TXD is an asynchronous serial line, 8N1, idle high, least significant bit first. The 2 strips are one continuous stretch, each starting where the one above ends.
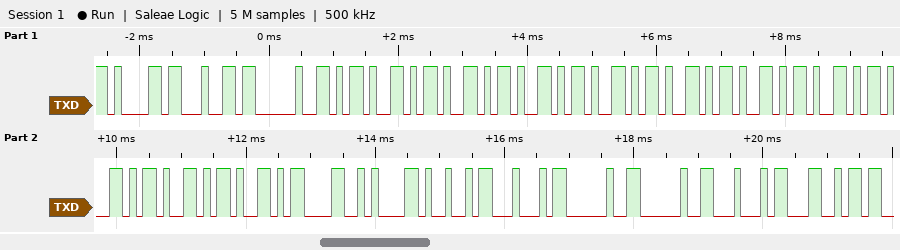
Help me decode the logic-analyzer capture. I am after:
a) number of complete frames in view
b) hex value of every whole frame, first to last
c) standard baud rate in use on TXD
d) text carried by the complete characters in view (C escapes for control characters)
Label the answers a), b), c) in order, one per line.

a) 21
b) 61 64 20 2D 2D 2D 2D 2D 2D 2D 2D 2D 2D 0D 0A 49 44 20 20 44 4C
c) 9600 baud
d) "ad ----------\r\nID  DL"
